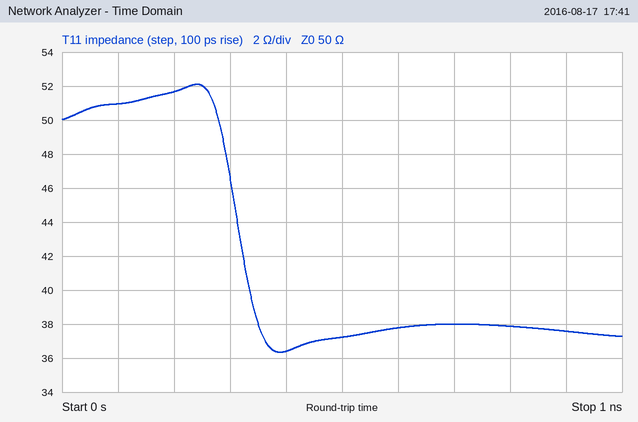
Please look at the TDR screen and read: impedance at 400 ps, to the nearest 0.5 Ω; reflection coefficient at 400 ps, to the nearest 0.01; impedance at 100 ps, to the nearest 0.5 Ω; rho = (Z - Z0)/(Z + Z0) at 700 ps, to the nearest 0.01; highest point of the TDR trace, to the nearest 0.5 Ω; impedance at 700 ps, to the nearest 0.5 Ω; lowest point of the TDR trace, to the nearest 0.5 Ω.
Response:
36.5 Ω
-0.16
51.0 Ω
-0.14
52.0 Ω
38.0 Ω
36.5 Ω
